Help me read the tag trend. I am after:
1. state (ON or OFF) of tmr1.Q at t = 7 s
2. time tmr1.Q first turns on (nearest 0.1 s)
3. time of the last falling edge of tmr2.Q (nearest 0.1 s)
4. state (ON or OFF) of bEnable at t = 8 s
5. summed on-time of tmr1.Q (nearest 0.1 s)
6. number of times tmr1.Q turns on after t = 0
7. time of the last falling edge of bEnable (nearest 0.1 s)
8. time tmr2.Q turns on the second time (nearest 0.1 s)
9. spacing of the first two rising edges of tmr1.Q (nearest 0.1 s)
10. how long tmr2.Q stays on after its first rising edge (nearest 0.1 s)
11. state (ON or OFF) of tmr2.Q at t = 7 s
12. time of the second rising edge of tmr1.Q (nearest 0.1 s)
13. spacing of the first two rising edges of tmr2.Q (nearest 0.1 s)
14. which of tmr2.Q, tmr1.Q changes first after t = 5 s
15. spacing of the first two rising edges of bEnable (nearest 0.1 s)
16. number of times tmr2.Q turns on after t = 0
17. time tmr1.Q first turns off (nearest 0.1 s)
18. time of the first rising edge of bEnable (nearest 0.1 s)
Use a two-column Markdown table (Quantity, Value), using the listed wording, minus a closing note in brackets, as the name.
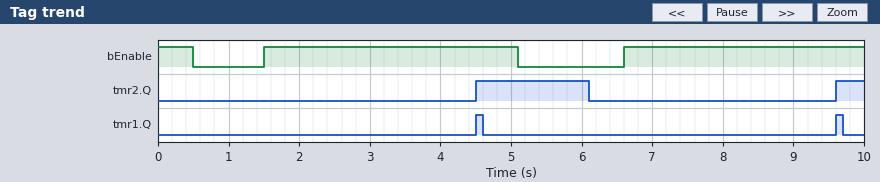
| Quantity | Value |
|---|---|
| state (ON or OFF) of tmr1.Q at t = 7 s | OFF |
| time tmr1.Q first turns on | 4.5 s |
| time of the last falling edge of tmr2.Q | 6.1 s |
| state (ON or OFF) of bEnable at t = 8 s | ON |
| summed on-time of tmr1.Q | 0.2 s |
| number of times tmr1.Q turns on after t = 0 | 2 |
| time of the last falling edge of bEnable | 5.1 s |
| time tmr2.Q turns on the second time | 9.6 s |
| spacing of the first two rising edges of tmr1.Q | 5.1 s |
| how long tmr2.Q stays on after its first rising edge | 1.6 s |
| state (ON or OFF) of tmr2.Q at t = 7 s | OFF |
| time of the second rising edge of tmr1.Q | 9.6 s |
| spacing of the first two rising edges of tmr2.Q | 5.1 s |
| which of tmr2.Q, tmr1.Q changes first after t = 5 s | tmr2.Q |
| spacing of the first two rising edges of bEnable | 5.1 s |
| number of times tmr2.Q turns on after t = 0 | 2 |
| time tmr1.Q first turns off | 4.6 s |
| time of the first rising edge of bEnable | 1.5 s |
